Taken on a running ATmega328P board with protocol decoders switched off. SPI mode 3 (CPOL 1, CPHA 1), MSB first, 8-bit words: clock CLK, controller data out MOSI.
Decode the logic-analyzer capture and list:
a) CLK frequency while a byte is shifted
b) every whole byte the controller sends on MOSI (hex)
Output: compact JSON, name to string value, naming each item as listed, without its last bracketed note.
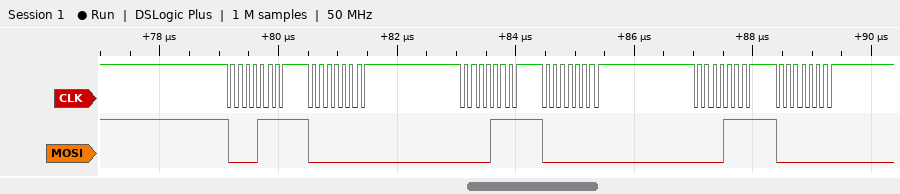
{"CLK frequency while a byte is shifted": "8 MHz", "every whole byte the controller sends on MOSI": "0F 00 0F 00 0F 00"}
